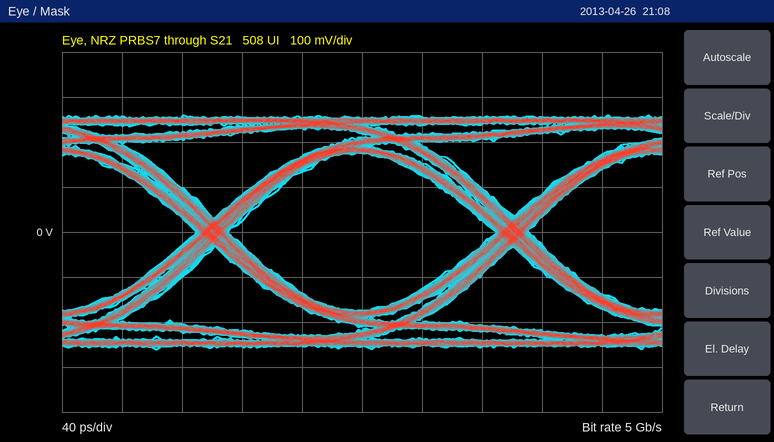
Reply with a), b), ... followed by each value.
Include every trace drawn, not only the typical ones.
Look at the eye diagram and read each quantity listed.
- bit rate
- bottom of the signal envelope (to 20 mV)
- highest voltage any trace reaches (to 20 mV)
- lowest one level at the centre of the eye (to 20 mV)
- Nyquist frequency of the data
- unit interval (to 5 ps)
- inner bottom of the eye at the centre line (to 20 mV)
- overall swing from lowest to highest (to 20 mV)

a) 5 Gb/s
b) -260 mV
c) 260 mV
d) 180 mV
e) 2.5 GHz
f) 200 ps
g) -180 mV
h) 520 mV
